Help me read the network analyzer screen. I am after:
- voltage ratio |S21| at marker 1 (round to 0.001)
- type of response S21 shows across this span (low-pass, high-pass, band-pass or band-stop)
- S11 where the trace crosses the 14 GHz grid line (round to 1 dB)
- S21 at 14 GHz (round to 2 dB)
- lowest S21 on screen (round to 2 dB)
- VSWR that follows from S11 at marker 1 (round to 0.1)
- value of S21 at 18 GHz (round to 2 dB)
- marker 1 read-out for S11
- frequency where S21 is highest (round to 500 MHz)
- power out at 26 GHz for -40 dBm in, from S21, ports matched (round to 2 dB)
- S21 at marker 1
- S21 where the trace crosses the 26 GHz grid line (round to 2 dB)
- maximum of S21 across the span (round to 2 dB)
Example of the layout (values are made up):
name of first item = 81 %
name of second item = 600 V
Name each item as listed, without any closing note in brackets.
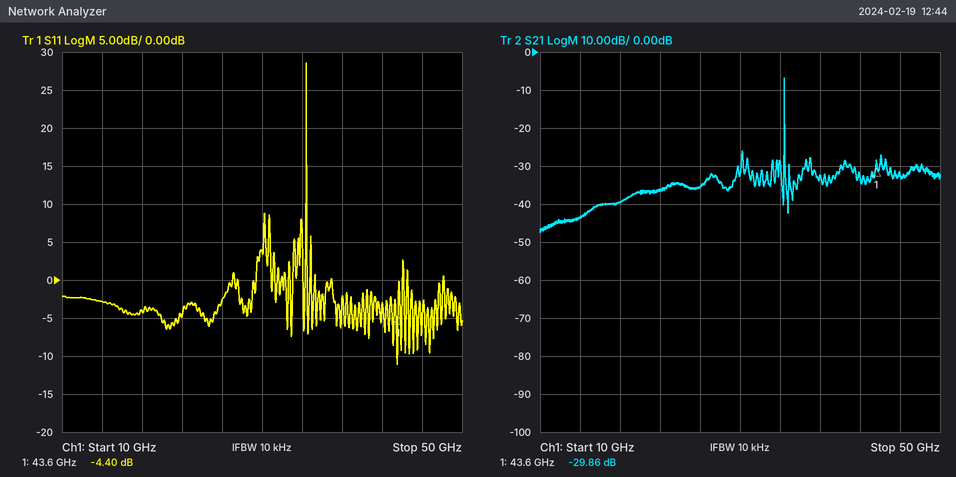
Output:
voltage ratio |S21| at marker 1 = 0.032
type of response S21 shows across this span = band-pass
S11 where the trace crosses the 14 GHz grid line = -3 dB
S21 at 14 GHz = -44 dB
lowest S21 on screen = -48 dB
VSWR that follows from S11 at marker 1 = 4.0
value of S21 at 18 GHz = -40 dB
marker 1 read-out for S11 = -4.40 dB
frequency where S21 is highest = 34.5 GHz
power out at 26 GHz for -40 dBm in, from S21, ports matched = -76 dBm
S21 at marker 1 = -29.86 dB
S21 where the trace crosses the 26 GHz grid line = -36 dB
maximum of S21 across the span = -6 dB
